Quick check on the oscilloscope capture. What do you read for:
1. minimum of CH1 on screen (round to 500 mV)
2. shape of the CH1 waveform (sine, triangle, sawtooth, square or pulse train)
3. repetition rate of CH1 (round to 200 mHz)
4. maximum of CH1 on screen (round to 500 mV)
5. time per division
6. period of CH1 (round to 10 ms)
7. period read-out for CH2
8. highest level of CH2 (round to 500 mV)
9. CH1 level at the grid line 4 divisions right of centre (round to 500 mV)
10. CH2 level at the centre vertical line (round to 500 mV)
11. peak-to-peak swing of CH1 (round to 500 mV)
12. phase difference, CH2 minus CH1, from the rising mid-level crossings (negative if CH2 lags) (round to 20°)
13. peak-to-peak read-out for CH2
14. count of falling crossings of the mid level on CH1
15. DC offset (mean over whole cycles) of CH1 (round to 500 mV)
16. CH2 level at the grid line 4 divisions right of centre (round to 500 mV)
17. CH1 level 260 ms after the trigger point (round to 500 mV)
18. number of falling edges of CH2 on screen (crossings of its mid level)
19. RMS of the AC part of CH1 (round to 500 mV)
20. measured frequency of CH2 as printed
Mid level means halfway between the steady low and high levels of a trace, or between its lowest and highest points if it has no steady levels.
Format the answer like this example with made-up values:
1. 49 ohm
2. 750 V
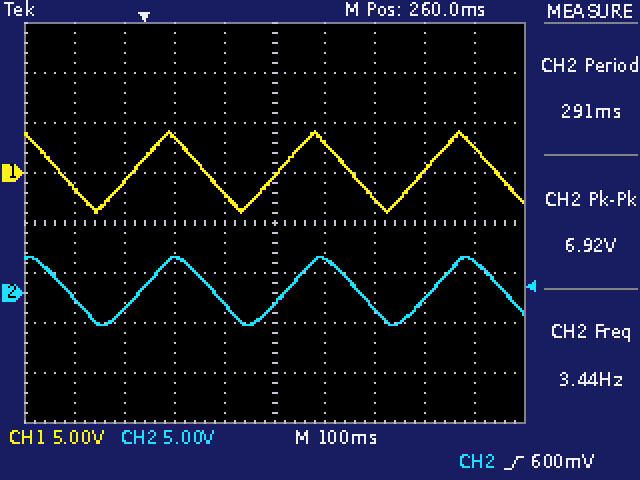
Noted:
1. -4.0 V
2. triangle
3. 3.4 Hz
4. 4.0 V
5. 100 ms
6. 290 ms
7. 291 ms
8. 3.5 V
9. 2.5 V
10. -1.0 V
11. 8.0 V
12. -20°
13. 6.92 V
14. 4
15. 0.0 V
16. 3.0 V
17. -500 mV
18. 4
19. 2.5 V
20. 3.44 Hz
